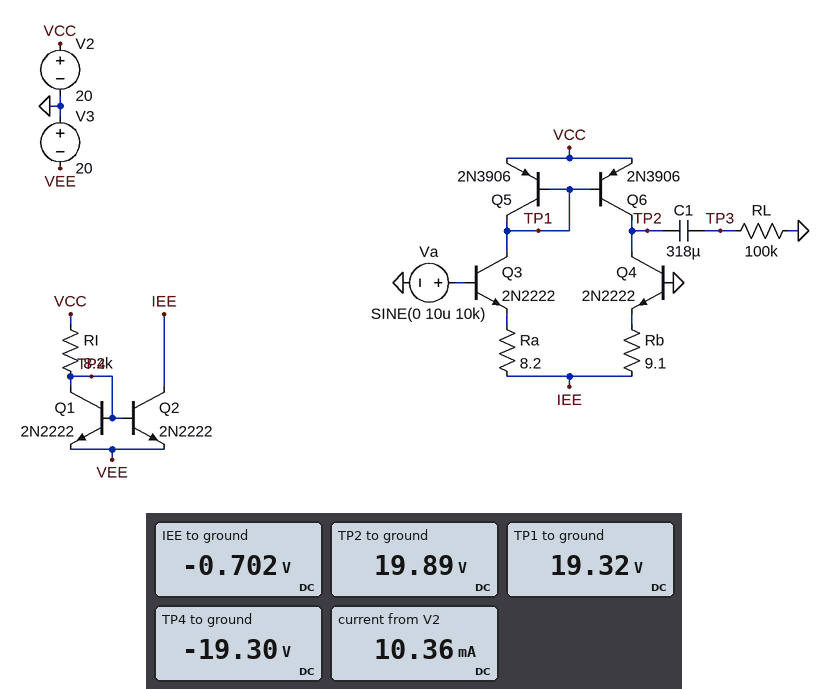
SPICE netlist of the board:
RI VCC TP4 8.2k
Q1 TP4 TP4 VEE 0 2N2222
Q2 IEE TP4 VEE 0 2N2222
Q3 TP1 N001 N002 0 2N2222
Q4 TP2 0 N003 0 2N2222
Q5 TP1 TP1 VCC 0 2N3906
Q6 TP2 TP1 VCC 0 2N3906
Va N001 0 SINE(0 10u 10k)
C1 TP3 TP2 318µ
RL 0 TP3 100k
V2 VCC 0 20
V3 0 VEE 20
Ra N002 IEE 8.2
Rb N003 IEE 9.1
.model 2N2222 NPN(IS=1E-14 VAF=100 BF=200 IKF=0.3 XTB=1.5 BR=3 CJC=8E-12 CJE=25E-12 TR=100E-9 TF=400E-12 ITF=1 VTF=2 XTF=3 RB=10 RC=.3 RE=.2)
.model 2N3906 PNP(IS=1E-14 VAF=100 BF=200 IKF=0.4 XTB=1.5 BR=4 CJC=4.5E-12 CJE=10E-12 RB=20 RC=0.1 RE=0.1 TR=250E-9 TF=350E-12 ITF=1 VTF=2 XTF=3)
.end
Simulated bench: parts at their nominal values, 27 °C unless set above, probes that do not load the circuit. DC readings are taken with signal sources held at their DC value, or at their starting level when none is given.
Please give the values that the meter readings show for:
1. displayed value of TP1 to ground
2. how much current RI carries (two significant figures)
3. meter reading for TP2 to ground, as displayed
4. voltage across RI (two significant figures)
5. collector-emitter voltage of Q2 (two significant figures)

19.32 V
4.8 mA
19.89 V
39 V
19 V
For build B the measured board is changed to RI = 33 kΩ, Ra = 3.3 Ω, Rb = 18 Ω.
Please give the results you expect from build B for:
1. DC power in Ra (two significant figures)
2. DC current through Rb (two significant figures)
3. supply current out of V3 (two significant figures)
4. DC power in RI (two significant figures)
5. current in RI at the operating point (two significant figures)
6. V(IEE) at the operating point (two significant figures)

2.1 µW
590 µA
2.6 mA
47 mW
1.2 mA
-650 mV
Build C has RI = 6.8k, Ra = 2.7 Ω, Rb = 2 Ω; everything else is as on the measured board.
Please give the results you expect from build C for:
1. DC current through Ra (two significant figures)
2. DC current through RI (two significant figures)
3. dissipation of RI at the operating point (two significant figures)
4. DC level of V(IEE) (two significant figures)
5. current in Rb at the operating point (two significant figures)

3.3 mA
5.8 mA
230 mW
-690 mV
3.4 mA
